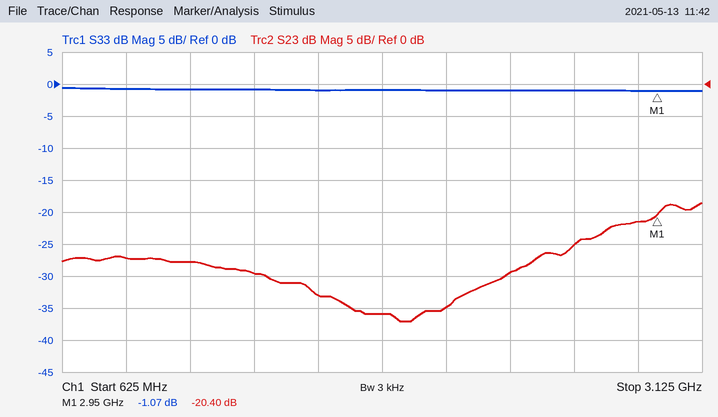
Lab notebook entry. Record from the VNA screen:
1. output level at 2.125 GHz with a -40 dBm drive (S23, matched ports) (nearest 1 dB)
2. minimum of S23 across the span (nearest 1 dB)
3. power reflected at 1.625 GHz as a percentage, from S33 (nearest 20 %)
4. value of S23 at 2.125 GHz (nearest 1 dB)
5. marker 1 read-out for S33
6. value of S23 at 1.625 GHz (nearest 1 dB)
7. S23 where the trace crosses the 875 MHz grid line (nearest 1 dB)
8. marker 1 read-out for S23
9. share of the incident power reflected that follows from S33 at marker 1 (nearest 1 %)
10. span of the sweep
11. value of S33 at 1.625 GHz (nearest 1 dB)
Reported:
-75 dBm
-37 dB
80 %
-35 dB
-1.07 dB
-33 dB
-27 dB
-20.40 dB
78 %
2.5 GHz
-1 dB
